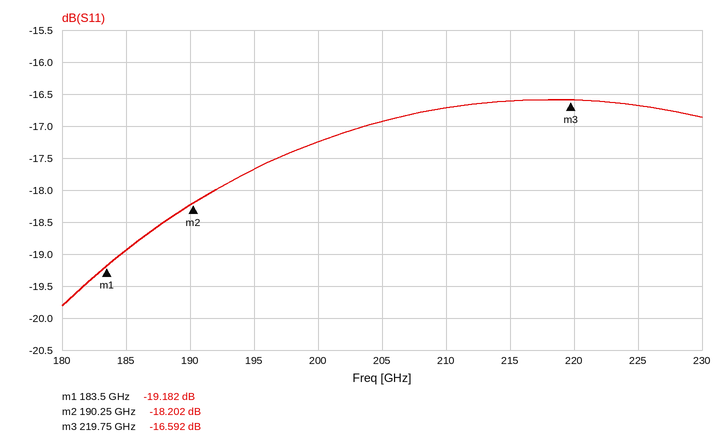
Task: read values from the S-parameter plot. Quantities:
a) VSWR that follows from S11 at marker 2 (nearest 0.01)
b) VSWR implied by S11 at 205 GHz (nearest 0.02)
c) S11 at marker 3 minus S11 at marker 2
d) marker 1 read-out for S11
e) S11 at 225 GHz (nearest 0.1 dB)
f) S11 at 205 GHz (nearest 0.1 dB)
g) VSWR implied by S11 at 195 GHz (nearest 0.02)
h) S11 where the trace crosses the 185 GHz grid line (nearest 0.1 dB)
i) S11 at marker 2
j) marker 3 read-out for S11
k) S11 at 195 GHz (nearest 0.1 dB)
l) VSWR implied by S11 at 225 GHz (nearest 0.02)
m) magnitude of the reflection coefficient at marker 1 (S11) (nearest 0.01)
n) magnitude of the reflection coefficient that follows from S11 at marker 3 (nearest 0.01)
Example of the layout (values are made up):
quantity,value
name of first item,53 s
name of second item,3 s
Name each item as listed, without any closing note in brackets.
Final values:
quantity,value
VSWR that follows from S11 at marker 2,1.28
VSWR implied by S11 at 205 GHz,1.34
S11 at marker 3 minus S11 at marker 2,1.610 dB
marker 1 read-out for S11,-19.182 dB
S11 at 225 GHz,-16.7 dB
S11 at 205 GHz,-16.9 dB
VSWR implied by S11 at 195 GHz,1.30
S11 where the trace crosses the 185 GHz grid line,-18.9 dB
S11 at marker 2,-18.202 dB
marker 3 read-out for S11,-16.592 dB
S11 at 195 GHz,-17.7 dB
VSWR implied by S11 at 225 GHz,1.34
magnitude of the reflection coefficient at marker 1 (S11),0.11
magnitude of the reflection coefficient that follows from S11 at marker 3,0.15
